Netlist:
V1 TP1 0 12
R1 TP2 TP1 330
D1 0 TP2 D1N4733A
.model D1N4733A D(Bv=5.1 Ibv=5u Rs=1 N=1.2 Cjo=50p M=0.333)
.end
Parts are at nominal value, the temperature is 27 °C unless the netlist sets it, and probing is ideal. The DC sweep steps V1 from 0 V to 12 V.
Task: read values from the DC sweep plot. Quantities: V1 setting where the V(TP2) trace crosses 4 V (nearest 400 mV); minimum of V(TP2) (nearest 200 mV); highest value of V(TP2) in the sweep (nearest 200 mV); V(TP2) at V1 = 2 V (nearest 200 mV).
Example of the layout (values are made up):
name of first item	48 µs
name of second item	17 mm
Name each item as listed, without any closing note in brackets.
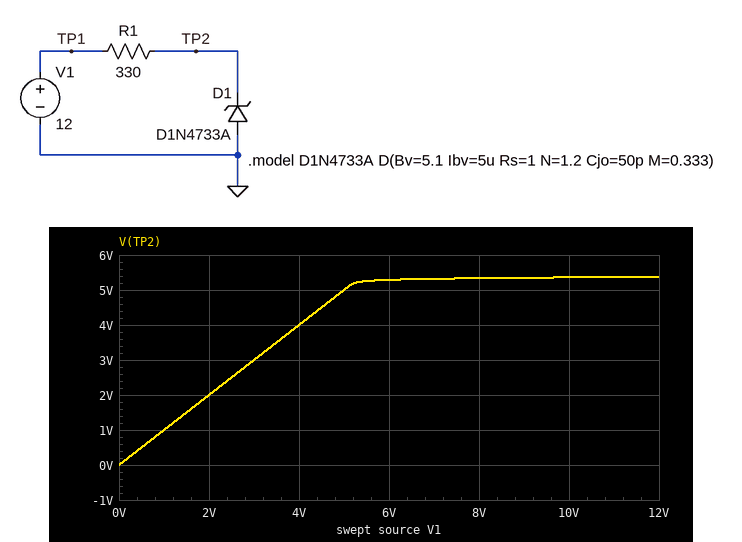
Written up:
V1 setting where the V(TP2) trace crosses 4 V	4.0 V
minimum of V(TP2)	0 V
highest value of V(TP2) in the sweep	5.4 V
V(TP2) at V1 = 2 V	2.0 V
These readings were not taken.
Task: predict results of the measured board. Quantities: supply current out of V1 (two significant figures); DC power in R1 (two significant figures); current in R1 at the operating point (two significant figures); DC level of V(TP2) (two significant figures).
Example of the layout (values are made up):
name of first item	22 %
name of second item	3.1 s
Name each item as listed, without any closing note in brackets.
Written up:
supply current out of V1	20 mA
DC power in R1	130 mW
current in R1 at the operating point	20 mA
DC level of V(TP2)	5.4 V
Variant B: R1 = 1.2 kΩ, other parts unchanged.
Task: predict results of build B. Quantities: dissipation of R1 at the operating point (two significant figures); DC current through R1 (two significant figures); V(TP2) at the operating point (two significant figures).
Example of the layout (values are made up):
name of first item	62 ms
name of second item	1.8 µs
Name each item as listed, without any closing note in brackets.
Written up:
dissipation of R1 at the operating point	37 mW
DC current through R1	5.6 mA
V(TP2) at the operating point	5.3 V
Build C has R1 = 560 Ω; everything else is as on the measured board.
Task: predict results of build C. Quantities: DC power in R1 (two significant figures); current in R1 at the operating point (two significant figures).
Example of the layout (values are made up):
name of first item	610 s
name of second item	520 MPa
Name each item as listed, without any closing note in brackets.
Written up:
DC power in R1	79 mW
current in R1 at the operating point	12 mA
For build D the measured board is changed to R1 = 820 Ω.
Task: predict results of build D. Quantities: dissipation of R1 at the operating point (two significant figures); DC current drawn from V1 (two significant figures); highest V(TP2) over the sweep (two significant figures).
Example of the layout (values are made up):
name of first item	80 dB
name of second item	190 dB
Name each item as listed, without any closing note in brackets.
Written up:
dissipation of R1 at the operating point	54 mW
DC current drawn from V1	8.1 mA
highest V(TP2) over the sweep	5.3 V
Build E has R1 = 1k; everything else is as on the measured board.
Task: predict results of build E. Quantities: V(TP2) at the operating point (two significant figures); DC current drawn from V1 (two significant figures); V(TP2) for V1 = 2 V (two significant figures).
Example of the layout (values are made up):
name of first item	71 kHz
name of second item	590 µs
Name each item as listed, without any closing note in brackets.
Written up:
V(TP2) at the operating point	5.3 V
DC current drawn from V1	6.7 mA
V(TP2) for V1 = 2 V	2.0 V
